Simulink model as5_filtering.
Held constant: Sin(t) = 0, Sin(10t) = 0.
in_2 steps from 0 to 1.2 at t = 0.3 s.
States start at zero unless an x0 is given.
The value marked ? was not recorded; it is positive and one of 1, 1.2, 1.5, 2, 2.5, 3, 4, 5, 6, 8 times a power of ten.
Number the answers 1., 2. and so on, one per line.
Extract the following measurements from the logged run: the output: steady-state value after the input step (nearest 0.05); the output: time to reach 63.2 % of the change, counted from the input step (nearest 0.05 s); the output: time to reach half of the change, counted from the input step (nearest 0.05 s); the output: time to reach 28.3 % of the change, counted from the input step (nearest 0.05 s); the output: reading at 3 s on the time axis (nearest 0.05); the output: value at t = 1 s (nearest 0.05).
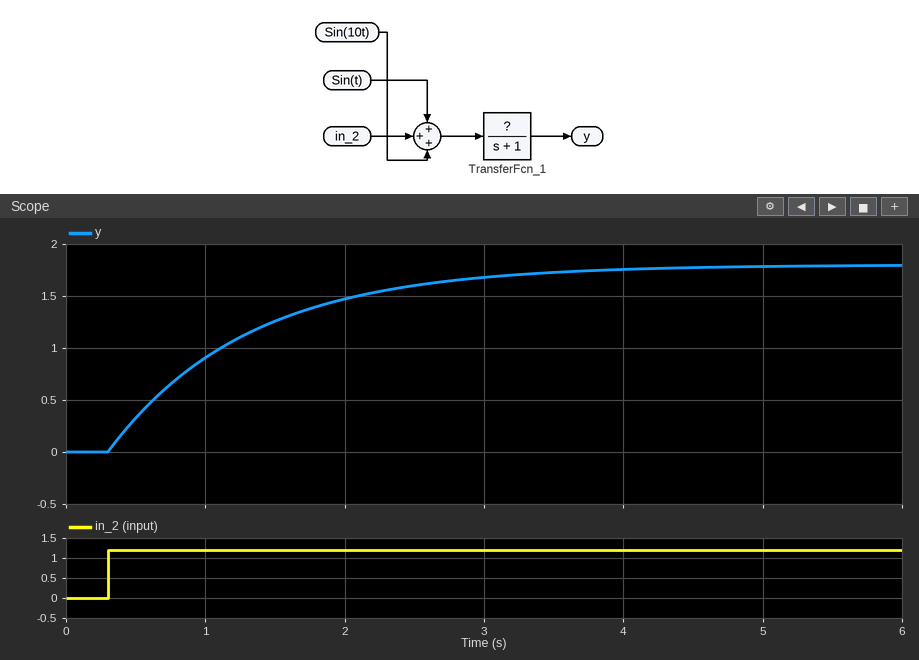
1. 1.80
2. 1.00 s
3. 0.70 s
4. 0.35 s
5. 1.70
6. 0.90
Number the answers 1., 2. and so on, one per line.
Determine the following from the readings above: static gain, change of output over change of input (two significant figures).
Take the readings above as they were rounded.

1. 1.5
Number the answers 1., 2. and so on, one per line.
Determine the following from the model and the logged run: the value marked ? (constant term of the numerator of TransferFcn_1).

1. 1.5
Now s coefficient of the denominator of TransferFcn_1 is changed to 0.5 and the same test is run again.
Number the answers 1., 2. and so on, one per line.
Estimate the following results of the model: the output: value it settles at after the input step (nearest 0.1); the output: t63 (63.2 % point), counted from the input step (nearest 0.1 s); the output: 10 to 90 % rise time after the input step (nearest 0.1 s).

1. 1.8
2. 0.5 s
3. 1.1 s
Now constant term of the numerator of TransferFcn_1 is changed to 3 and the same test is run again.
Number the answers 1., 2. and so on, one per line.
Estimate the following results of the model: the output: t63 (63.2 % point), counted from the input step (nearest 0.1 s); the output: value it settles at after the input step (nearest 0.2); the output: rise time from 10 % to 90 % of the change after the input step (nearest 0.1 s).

1. 1.0 s
2. 3.6
3. 2.2 s
